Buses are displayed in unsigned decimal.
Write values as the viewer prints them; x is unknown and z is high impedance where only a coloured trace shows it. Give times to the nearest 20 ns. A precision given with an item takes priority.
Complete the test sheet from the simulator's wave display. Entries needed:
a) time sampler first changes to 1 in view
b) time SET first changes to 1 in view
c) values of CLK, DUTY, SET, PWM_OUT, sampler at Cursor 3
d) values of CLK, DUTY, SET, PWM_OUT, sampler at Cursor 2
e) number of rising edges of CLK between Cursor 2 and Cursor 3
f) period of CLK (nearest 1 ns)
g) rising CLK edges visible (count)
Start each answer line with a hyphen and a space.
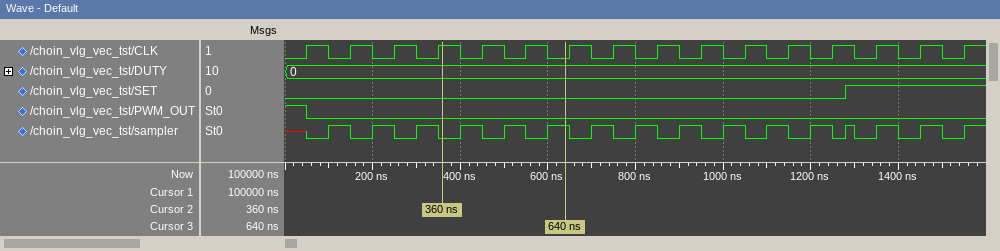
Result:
- 100 ns
- 1280 ns
- CLK=0, DUTY=0, SET=0, PWM_OUT=0, sampler=1
- CLK=1, DUTY=0, SET=0, PWM_OUT=0, sampler=0
- 2
- 100 ns
- 16
